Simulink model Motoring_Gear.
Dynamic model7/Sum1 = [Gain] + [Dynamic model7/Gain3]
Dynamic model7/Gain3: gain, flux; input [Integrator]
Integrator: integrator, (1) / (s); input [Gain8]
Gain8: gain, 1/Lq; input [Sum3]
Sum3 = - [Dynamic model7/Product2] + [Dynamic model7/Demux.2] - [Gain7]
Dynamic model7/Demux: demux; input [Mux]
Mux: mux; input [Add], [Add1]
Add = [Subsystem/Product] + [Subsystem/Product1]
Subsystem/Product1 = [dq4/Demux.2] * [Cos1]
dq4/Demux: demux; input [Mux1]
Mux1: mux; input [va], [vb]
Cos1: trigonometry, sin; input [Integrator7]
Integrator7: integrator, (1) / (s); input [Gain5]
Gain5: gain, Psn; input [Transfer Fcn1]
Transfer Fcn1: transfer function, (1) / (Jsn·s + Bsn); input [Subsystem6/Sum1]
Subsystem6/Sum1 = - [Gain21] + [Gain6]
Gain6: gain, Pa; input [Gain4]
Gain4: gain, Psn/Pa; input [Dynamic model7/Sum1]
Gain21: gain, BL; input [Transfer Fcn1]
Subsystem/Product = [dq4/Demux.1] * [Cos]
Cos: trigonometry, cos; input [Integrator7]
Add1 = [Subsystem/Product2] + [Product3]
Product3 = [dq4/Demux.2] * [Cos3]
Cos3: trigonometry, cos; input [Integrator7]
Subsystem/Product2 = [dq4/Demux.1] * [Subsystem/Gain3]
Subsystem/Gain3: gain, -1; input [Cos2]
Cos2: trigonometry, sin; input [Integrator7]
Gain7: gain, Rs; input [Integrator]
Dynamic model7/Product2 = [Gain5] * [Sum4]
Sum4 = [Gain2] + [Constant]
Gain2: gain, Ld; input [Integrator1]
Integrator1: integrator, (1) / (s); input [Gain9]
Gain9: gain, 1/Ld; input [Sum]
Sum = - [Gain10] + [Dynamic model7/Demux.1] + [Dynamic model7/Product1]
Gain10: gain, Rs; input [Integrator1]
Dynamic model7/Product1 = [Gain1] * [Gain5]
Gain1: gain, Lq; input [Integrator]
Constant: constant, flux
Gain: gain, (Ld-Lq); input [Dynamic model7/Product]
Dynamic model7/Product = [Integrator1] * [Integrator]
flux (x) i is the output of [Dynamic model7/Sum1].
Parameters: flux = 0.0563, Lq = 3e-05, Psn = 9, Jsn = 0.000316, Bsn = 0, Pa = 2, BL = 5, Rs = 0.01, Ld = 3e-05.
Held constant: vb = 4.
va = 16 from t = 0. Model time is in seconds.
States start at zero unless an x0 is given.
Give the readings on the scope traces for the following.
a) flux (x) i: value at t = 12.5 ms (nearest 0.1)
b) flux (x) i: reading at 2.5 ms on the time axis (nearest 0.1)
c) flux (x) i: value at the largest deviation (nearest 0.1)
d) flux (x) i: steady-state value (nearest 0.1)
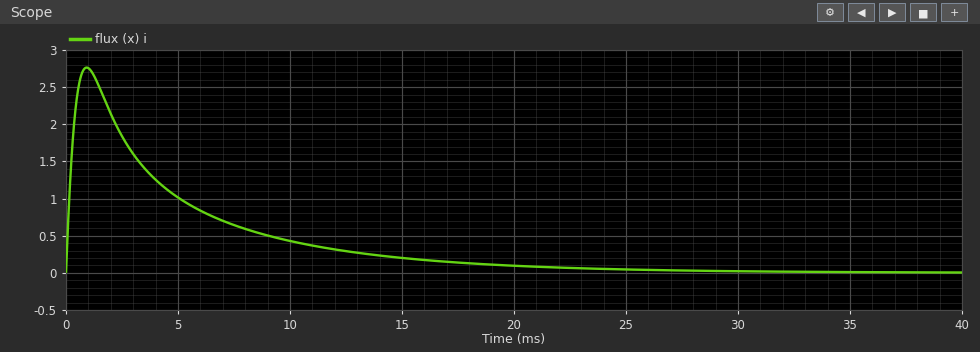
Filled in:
0.3
1.8
2.8
0.0
